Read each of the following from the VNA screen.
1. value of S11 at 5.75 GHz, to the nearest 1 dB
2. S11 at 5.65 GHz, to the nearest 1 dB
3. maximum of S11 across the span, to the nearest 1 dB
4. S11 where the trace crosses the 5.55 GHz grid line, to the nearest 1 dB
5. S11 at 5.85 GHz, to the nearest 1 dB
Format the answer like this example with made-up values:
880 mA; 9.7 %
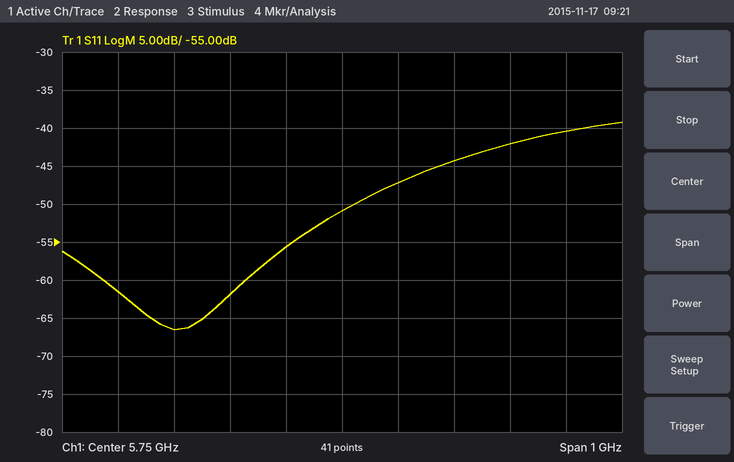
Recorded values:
-51 dB; -56 dB; -39 dB; -62 dB; -47 dB
